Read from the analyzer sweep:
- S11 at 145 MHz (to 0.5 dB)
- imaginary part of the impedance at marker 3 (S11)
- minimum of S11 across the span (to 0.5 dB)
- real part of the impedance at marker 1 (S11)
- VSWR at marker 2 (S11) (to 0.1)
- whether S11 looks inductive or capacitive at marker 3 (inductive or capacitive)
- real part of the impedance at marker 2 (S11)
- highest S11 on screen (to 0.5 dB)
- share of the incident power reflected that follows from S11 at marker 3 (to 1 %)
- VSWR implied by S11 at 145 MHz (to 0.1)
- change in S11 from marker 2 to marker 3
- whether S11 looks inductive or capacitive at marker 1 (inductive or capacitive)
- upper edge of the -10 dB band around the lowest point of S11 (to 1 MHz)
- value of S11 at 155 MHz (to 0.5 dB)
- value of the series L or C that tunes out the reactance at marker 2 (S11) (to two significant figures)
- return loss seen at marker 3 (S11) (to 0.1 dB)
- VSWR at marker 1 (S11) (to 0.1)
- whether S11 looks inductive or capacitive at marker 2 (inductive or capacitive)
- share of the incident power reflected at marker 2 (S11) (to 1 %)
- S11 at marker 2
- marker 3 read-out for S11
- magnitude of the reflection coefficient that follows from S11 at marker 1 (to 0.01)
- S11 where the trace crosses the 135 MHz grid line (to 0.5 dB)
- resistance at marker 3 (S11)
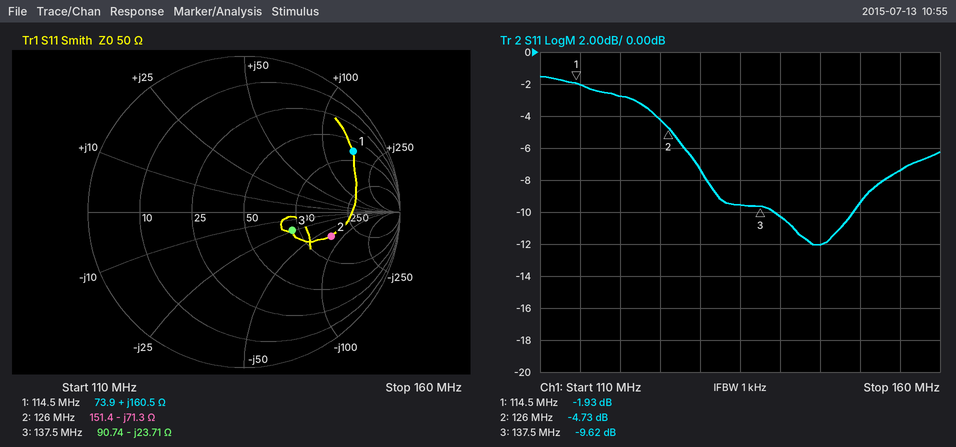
-12.0 dB
-23.71 Ω
-12.0 dB
73.9 Ω
3.8
capacitive
151.4 Ω
-1.5 dB
11 %
1.7
-4.89 dB
inductive
149 MHz
-7.5 dB
90 nH
9.6 dB
9.0
capacitive
34 %
-4.73 dB
-9.62 dB
0.80
-9.5 dB
90.74 Ω
